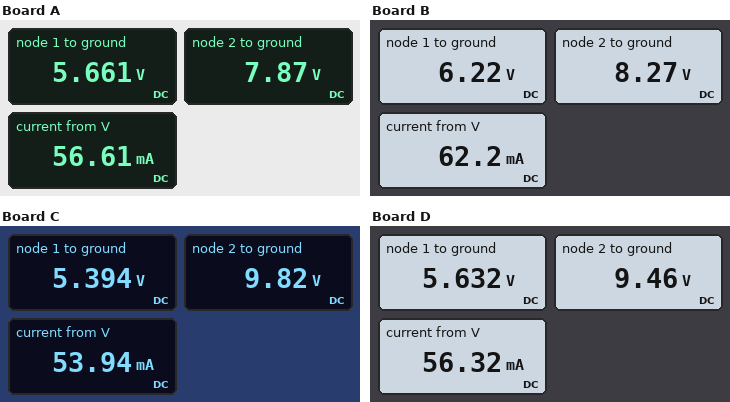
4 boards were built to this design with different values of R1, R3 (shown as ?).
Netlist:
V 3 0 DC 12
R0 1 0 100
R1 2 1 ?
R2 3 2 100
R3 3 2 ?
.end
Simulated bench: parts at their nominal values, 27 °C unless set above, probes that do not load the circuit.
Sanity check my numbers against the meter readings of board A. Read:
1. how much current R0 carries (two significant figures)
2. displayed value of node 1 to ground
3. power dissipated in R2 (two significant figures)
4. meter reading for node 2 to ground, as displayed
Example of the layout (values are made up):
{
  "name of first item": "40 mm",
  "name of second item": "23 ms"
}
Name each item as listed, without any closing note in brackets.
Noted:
{
  "how much current R0 carries": "57 mA",
  "displayed value of node 1 to ground": "5.661 V",
  "power dissipated in R2": "170 mW",
  "meter reading for node 2 to ground, as displayed": "7.87 V"
}
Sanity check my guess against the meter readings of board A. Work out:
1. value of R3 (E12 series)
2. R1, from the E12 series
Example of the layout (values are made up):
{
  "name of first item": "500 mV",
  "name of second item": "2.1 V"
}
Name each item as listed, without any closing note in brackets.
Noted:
{
  "value of R3": "270 Ω",
  "R1, from the E12 series": "39 Ω"
}
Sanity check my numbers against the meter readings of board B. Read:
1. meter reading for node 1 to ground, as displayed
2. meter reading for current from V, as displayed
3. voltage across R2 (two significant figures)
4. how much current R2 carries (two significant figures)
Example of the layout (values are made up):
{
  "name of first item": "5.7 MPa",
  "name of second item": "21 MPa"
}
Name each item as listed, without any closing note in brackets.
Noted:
{
  "meter reading for node 1 to ground, as displayed": "6.22 V",
  "meter reading for current from V, as displayed": "62.2 mA",
  "voltage across R2": "3.7 V",
  "how much current R2 carries": "37 mA"
}
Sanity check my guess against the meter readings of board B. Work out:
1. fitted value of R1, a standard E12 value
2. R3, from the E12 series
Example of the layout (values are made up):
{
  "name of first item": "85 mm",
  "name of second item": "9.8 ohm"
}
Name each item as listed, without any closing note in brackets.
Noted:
{
  "fitted value of R1, a standard E12 value": "33 Ω",
  "R3, from the E12 series": "150 Ω"
}
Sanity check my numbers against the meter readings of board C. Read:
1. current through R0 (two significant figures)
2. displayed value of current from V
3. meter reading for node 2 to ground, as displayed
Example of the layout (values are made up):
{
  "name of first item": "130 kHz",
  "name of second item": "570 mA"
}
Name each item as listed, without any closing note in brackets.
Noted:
{
  "current through R0": "54 mA",
  "displayed value of current from V": "53.94 mA",
  "meter reading for node 2 to ground, as displayed": "9.82 V"
}
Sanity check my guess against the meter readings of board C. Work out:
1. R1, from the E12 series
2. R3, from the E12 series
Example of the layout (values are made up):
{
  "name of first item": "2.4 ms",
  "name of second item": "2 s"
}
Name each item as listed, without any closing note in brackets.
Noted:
{
  "R1, from the E12 series": "82 Ω",
  "R3, from the E12 series": "68 Ω"
}
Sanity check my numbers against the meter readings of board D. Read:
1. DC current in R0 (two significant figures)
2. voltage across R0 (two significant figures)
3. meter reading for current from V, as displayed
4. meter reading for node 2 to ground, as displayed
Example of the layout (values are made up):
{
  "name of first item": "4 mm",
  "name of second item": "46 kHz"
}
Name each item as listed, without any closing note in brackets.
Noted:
{
  "DC current in R0": "56 mA",
  "voltage across R0": "5.6 V",
  "meter reading for current from V, as displayed": "56.32 mA",
  "meter reading for node 2 to ground, as displayed": "9.46 V"
}
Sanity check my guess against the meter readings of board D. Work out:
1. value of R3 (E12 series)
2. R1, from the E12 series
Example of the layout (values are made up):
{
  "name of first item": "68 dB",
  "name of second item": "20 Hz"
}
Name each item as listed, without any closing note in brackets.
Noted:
{
  "value of R3": "82 Ω",
  "R1, from the E12 series": "68 Ω"
}
